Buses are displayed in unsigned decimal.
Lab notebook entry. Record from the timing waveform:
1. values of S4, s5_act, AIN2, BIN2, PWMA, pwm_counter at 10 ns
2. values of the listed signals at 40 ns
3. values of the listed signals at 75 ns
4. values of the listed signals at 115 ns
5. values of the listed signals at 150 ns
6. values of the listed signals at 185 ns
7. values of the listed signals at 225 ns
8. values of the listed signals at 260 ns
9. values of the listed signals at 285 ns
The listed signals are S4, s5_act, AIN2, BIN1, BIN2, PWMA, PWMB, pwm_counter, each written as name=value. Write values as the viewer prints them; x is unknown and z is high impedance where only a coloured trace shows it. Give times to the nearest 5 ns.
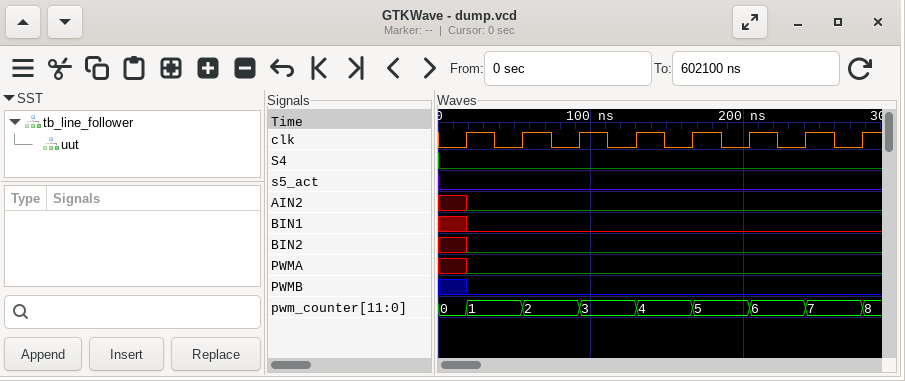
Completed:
S4=0, s5_act=0, AIN2=x, BIN2=x, PWMA=x, pwm_counter=0
S4=0, s5_act=0, AIN2=0, BIN1=0, BIN2=0, PWMA=0, PWMB=0, pwm_counter=1
S4=0, s5_act=0, AIN2=0, BIN1=0, BIN2=0, PWMA=0, PWMB=0, pwm_counter=2
S4=0, s5_act=0, AIN2=0, BIN1=0, BIN2=0, PWMA=0, PWMB=0, pwm_counter=3
S4=0, s5_act=0, AIN2=0, BIN1=0, BIN2=0, PWMA=0, PWMB=0, pwm_counter=4
S4=0, s5_act=0, AIN2=0, BIN1=0, BIN2=0, PWMA=0, PWMB=0, pwm_counter=5
S4=0, s5_act=0, AIN2=0, BIN1=0, BIN2=0, PWMA=0, PWMB=0, pwm_counter=6
S4=0, s5_act=0, AIN2=0, BIN1=0, BIN2=0, PWMA=0, PWMB=0, pwm_counter=7
S4=0, s5_act=0, AIN2=0, BIN1=0, BIN2=0, PWMA=0, PWMB=0, pwm_counter=8
